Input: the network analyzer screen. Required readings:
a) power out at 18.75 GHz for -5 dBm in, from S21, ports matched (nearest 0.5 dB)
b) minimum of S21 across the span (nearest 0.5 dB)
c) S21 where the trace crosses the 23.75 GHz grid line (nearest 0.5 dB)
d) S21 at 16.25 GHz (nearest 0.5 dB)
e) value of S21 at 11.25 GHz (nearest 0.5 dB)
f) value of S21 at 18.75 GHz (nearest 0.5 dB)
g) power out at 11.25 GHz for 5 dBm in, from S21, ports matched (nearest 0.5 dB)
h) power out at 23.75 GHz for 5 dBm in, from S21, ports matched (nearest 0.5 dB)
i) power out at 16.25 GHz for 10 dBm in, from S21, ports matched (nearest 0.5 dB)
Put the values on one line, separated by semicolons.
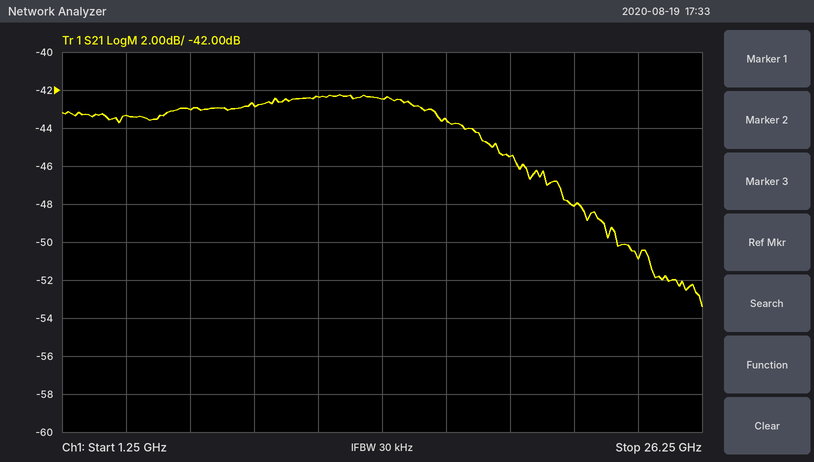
-50.5 dBm; -53.5 dB; -51.0 dB; -43.5 dB; -42.5 dB; -45.5 dB; -37.5 dBm; -46.0 dBm; -33.5 dBm
